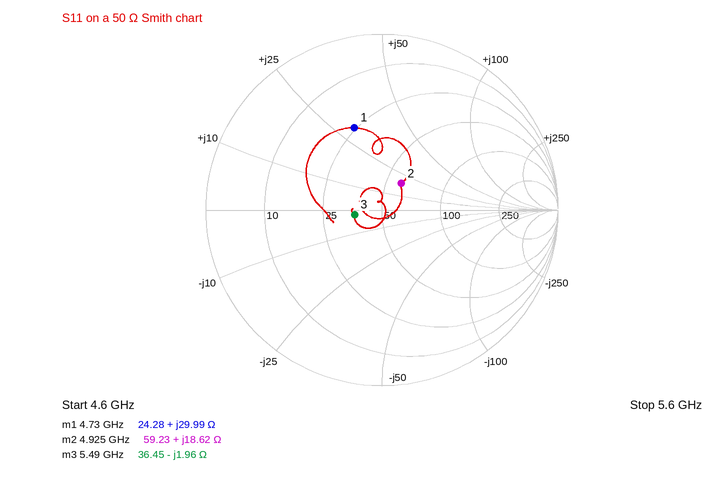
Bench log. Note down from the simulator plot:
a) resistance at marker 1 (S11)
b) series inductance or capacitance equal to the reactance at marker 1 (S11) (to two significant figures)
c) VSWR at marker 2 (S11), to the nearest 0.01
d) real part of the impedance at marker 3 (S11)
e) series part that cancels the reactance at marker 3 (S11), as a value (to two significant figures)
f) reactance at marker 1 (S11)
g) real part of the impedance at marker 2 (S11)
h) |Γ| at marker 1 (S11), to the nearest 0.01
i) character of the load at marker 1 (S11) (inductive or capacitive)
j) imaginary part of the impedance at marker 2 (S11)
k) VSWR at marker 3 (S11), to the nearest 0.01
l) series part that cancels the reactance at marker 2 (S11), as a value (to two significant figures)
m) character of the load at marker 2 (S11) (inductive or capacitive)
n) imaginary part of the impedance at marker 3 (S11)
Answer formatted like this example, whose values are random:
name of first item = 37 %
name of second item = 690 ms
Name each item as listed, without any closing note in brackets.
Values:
resistance at marker 1 = 24.28 Ω
series inductance or capacitance equal to the reactance at marker 1 (S11) = 1.0 nH
VSWR at marker 2 (S11), to the nearest 0.01 = 1.46
real part of the impedance at marker 3 = 36.45 Ω
series part that cancels the reactance at marker 3 (S11), as a value = 57 pH
reactance at marker 1 = +29.99 Ω
real part of the impedance at marker 2 = 59.23 Ω
|Γ| at marker 1 (S11), to the nearest 0.01 = 0.49
character of the load at marker 1 (S11) = inductive
imaginary part of the impedance at marker 2 = +18.62 Ω
VSWR at marker 3 (S11), to the nearest 0.01 = 1.38
series part that cancels the reactance at marker 2 (S11), as a value = 1.7 pF
character of the load at marker 2 (S11) = inductive
imaginary part of the impedance at marker 3 = -1.96 Ω
